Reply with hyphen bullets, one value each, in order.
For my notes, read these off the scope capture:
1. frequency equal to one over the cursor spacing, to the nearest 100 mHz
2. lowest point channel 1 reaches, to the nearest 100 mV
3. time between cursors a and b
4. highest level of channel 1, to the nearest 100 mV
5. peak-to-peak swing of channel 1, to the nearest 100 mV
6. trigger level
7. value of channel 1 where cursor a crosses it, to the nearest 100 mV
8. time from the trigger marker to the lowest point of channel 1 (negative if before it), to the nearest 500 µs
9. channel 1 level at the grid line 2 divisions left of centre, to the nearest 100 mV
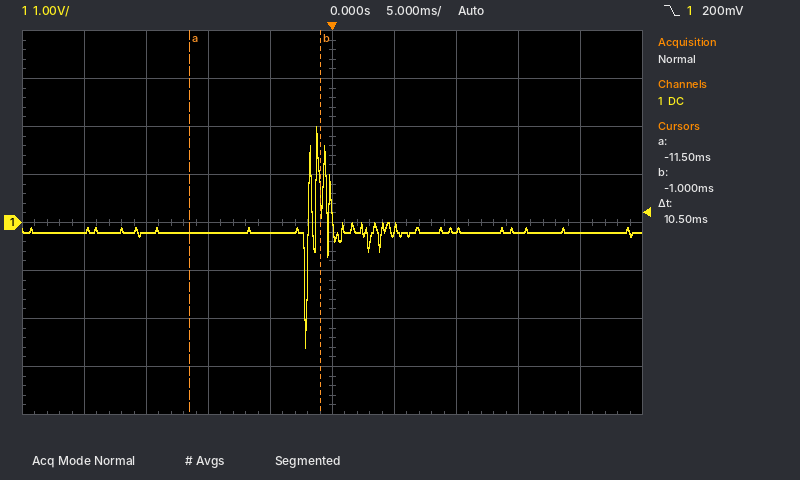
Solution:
- 95.2 Hz
- -2.6 V
- 10.5 ms
- 2.0 V
- 4.6 V
- 200 mV
- -200 mV
- -2.0 ms
- -200 mV
